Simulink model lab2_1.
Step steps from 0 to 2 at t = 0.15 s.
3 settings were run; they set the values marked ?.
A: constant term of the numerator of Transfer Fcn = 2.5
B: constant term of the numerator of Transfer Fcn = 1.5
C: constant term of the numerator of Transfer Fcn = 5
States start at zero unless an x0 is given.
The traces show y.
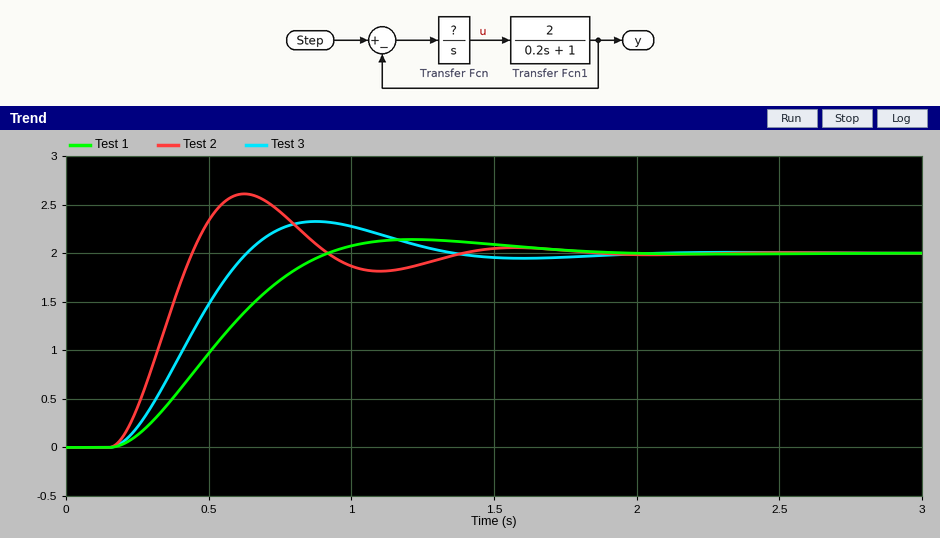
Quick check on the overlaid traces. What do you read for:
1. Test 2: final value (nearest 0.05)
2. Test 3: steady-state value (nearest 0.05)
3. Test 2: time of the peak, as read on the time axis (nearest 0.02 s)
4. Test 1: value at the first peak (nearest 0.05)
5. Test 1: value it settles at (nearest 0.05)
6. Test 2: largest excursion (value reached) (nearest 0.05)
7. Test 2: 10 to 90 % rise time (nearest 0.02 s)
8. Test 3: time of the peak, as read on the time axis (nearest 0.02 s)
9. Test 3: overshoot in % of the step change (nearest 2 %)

2.00
2.00
0.62 s
2.15
2.00
2.60
0.20 s
0.88 s
16 %
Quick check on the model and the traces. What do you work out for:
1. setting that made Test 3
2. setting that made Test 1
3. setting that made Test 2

A
B
C
